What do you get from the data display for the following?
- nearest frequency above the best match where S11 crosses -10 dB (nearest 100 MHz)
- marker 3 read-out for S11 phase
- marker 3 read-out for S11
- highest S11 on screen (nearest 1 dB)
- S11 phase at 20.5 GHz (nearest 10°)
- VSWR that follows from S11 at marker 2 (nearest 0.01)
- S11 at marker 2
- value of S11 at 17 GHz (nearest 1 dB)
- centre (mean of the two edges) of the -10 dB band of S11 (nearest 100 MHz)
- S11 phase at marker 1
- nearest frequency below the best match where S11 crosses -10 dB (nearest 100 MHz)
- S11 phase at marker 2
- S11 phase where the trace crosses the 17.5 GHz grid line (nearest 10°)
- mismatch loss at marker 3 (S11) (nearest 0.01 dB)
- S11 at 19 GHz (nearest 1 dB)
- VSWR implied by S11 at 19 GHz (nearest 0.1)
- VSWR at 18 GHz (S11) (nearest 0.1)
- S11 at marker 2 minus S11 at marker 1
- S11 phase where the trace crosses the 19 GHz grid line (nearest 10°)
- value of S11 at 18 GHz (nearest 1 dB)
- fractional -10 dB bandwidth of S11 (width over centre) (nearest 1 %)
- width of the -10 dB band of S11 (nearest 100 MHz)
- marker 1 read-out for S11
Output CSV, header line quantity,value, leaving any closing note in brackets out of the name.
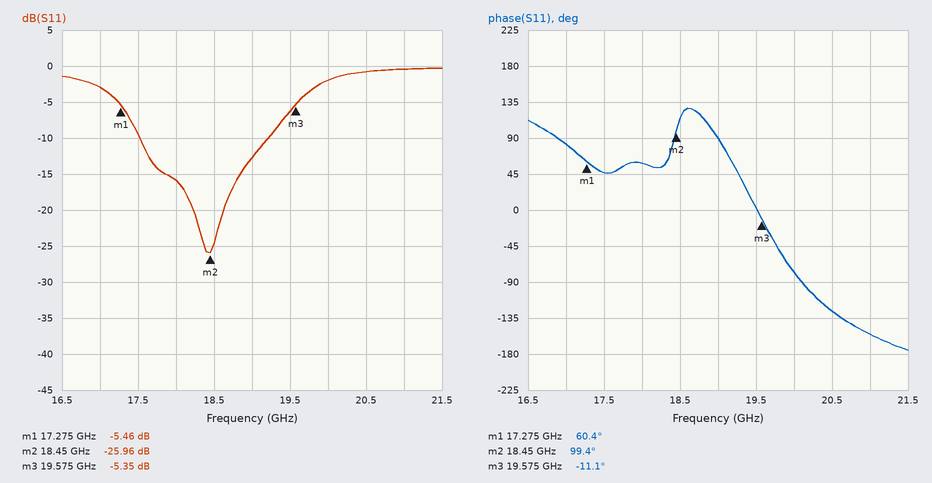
quantity,value
nearest frequency above the best match where S11 crosses -10 dB,19.2 GHz
marker 3 read-out for S11 phase,-11.1°
marker 3 read-out for S11,-5.35 dB
highest S11 on screen,0 dB
S11 phase at 20.5 GHz,-130°
VSWR that follows from S11 at marker 2,1.11
S11 at marker 2,-25.96 dB
value of S11 at 17 GHz,-3 dB
centre (mean of the two edges) of the -10 dB band of S11,18.4 GHz
S11 phase at marker 1,60.4°
nearest frequency below the best match where S11 crosses -10 dB,17.5 GHz
S11 phase at marker 2,99.4°
S11 phase where the trace crosses the 17.5 GHz grid line,50°
mismatch loss at marker 3 (S11),1.50 dB
S11 at 19 GHz,-13 dB
VSWR implied by S11 at 19 GHz,1.6
VSWR at 18 GHz (S11),1.4
S11 at marker 2 minus S11 at marker 1,-20.50 dB
S11 phase where the trace crosses the 19 GHz grid line,90°
value of S11 at 18 GHz,-16 dB
fractional -10 dB bandwidth of S11 (width over centre),9 %
width of the -10 dB band of S11,1.7 GHz
marker 1 read-out for S11,-5.46 dB
